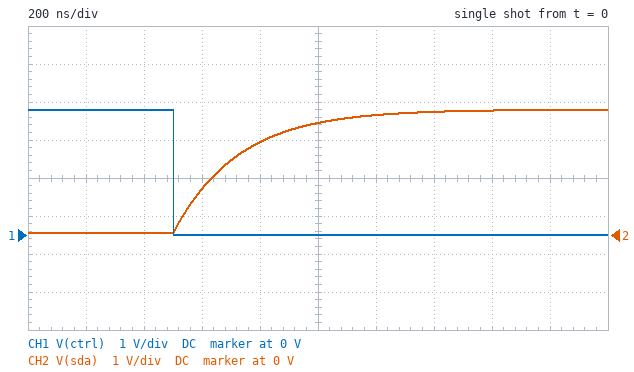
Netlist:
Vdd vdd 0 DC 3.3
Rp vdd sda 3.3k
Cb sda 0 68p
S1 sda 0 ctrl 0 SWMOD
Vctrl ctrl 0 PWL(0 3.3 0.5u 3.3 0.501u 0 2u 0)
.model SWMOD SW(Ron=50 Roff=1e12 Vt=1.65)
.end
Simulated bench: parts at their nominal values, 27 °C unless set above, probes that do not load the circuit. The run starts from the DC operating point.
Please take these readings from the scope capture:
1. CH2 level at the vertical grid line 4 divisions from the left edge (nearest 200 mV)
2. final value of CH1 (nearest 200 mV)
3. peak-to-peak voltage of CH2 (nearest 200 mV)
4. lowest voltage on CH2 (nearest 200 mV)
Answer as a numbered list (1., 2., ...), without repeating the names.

1. 2.4 V
2. 0 V
3. 3.2 V
4. 0 V
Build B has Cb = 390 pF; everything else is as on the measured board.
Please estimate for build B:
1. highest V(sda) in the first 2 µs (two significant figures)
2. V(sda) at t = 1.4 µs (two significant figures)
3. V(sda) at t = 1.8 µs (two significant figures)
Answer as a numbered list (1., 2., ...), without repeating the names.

1. 2.3 V
2. 1.7 V
3. 2.1 V
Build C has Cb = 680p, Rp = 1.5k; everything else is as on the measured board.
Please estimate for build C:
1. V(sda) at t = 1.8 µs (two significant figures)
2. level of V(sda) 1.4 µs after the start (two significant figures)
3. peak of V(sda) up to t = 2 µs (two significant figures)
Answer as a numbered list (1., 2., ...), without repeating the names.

1. 2.4 V
2. 2.0 V
3. 2.6 V
